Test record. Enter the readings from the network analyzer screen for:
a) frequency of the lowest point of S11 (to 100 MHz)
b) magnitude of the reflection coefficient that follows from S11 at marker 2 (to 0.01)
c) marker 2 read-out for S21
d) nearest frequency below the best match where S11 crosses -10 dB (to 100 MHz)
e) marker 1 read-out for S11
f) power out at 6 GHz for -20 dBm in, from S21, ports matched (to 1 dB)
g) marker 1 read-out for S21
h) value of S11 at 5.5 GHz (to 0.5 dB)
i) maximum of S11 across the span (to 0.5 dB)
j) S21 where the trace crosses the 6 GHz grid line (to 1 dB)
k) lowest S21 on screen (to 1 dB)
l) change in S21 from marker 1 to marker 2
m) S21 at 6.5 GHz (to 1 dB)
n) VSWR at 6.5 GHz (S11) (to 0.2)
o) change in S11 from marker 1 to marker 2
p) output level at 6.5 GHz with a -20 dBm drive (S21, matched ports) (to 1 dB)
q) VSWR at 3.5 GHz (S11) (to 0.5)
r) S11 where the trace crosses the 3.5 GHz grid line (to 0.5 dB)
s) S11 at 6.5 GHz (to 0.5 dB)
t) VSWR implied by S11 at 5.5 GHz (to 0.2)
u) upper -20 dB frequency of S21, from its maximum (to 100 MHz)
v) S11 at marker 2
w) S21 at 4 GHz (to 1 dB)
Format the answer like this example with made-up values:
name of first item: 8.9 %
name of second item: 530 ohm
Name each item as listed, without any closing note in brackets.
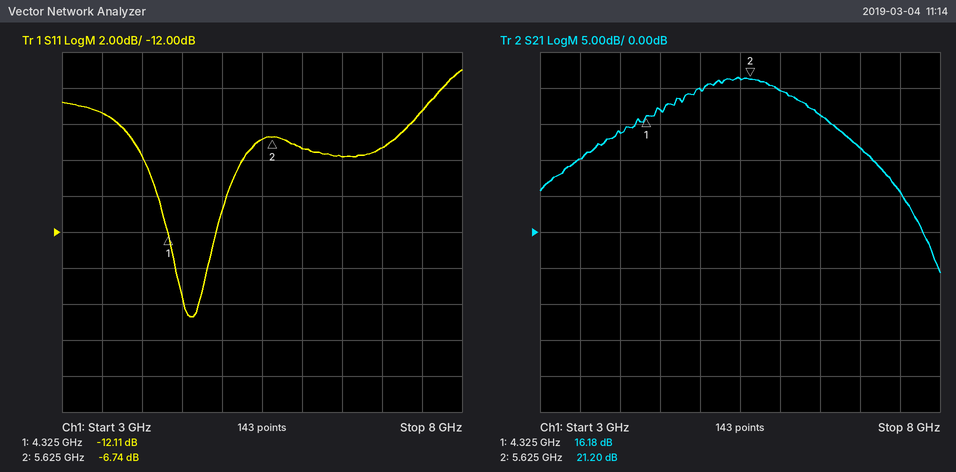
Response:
frequency of the lowest point of S11: 4.6 GHz
magnitude of the reflection coefficient that follows from S11 at marker 2: 0.46
marker 2 read-out for S21: 21.20 dB
nearest frequency below the best match where S11 crosses -10 dB: 4.2 GHz
marker 1 read-out for S11: -12.11 dB
power out at 6 GHz for -20 dBm in, from S21, ports matched: 0 dBm
marker 1 read-out for S21: 16.18 dB
value of S11 at 5.5 GHz: -7.0 dB
maximum of S11 across the span: -3.0 dB
S21 where the trace crosses the 6 GHz grid line: 20 dB
lowest S21 on screen: -6 dB
change in S21 from marker 1 to marker 2: 5.02 dB
S21 at 6.5 GHz: 16 dB
VSWR at 6.5 GHz (S11): 2.4
change in S11 from marker 1 to marker 2: 5.37 dB
output level at 6.5 GHz with a -20 dBm drive (S21, matched ports): -4 dBm
VSWR at 3.5 GHz (S11): 3.5
S11 where the trace crosses the 3.5 GHz grid line: -5.5 dB
S11 at 6.5 GHz: -8.0 dB
VSWR implied by S11 at 5.5 GHz: 2.6
upper -20 dB frequency of S21, from its maximum: 7.7 GHz
S11 at marker 2: -6.74 dB
S21 at 4 GHz: 14 dB
